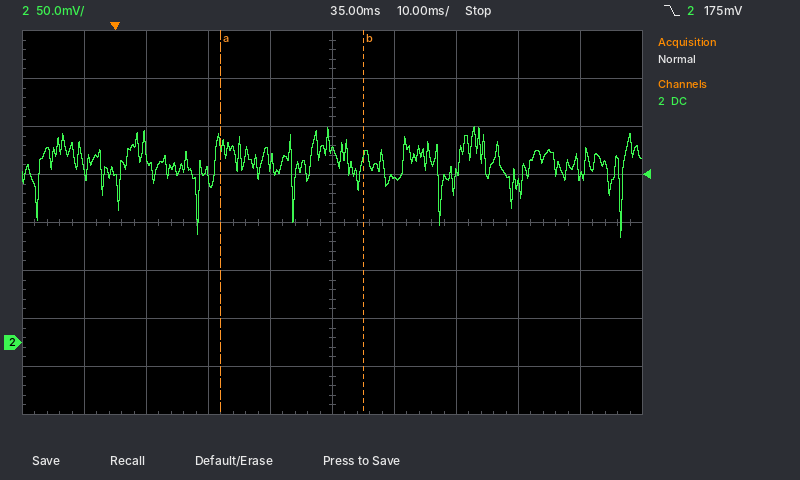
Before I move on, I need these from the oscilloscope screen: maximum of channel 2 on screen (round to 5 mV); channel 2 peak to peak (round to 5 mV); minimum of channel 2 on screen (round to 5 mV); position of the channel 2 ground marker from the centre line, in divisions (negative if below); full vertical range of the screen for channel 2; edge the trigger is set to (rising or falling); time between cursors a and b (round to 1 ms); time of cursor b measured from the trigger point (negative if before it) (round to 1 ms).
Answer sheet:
225 mV
115 mV
110 mV
-2.5 div
400 mV
falling
23 ms
+40 ms
